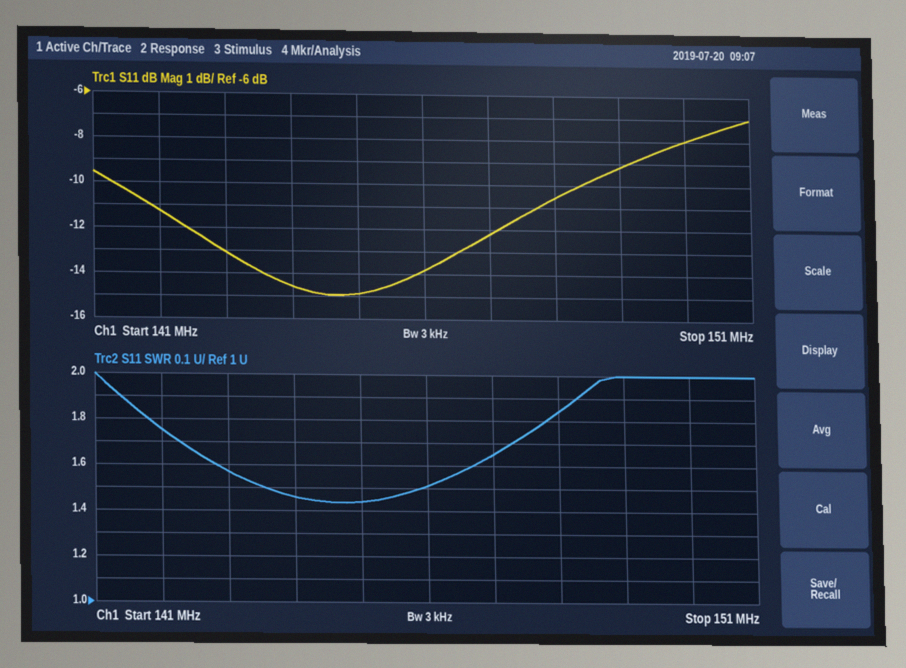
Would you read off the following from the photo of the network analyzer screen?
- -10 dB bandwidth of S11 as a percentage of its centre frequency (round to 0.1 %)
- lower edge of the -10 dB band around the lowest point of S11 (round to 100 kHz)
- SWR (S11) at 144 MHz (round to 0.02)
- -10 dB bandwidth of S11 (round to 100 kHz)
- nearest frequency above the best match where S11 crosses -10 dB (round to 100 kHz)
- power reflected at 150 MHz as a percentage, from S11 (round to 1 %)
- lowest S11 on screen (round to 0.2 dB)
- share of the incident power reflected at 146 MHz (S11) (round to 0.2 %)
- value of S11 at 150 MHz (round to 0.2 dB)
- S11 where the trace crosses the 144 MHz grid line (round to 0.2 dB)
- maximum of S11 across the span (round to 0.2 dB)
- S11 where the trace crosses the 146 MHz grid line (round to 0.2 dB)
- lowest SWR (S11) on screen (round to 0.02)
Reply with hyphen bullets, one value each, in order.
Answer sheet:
- 4.9 %
- 141.3 MHz
- 1.46
- 7.1 MHz
- 148.4 MHz
- 16 %
- -15.0 dB
- 4.2 %
- -8.0 dB
- -14.6 dB
- -7.0 dB
- -13.8 dB
- 1.44
